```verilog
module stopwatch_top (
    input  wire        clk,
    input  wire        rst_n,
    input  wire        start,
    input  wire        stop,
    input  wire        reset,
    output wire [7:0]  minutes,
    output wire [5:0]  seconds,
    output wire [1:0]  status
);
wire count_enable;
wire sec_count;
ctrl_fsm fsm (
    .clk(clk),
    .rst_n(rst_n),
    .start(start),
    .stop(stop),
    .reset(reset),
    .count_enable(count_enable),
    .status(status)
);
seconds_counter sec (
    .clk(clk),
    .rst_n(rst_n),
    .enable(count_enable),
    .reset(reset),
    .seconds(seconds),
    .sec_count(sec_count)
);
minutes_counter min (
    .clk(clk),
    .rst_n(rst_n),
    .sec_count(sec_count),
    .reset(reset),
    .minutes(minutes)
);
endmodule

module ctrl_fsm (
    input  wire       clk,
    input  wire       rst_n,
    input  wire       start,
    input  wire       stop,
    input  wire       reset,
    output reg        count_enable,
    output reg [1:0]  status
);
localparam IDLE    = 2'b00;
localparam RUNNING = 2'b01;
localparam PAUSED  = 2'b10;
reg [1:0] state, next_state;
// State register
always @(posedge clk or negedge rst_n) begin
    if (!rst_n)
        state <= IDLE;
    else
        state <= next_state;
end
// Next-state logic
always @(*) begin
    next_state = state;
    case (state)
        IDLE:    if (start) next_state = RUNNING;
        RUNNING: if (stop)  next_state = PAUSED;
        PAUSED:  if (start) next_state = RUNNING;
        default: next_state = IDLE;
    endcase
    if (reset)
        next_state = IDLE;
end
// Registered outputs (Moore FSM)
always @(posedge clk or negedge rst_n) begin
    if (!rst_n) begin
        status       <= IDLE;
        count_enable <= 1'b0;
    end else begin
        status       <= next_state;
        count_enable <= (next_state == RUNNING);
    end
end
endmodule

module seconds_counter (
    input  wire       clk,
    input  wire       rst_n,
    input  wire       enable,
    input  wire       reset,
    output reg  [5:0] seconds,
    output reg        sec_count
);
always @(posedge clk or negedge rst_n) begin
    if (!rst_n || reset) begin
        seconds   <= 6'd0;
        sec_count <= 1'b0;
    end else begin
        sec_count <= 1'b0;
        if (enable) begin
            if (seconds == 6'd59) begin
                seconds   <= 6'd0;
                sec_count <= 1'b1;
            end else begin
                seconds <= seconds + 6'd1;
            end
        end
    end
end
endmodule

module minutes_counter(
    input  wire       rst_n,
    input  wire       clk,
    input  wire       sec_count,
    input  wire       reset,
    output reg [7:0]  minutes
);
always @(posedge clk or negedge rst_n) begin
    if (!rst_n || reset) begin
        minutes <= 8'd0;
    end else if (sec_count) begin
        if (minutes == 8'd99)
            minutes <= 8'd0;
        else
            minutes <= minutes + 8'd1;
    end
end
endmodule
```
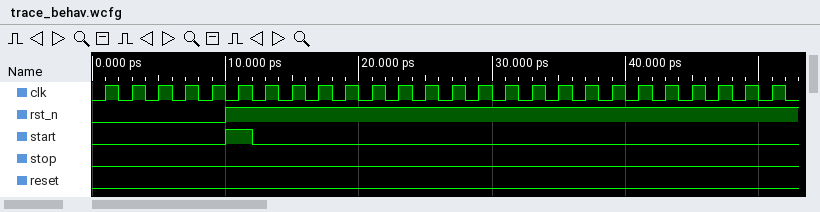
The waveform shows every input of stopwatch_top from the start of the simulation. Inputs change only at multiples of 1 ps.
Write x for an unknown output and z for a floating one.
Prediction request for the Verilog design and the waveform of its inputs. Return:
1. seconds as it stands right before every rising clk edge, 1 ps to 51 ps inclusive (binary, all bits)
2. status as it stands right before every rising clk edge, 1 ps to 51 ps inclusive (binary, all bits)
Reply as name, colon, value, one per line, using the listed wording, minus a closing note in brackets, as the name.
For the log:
seconds as it stands right before every rising clk edge, 1 ps to 51 ps inclusive: 000000, 000000, 000000, 000000, 000000, 000000, 000000, 000001, 000010, 000011, 000100, 000101, 000110, 000111, 001000, 001001, 001010, 001011, 001100, 001101, 001110, 001111, 010000, 010001, 010010, 010011
status as it stands right before every rising clk edge, 1 ps to 51 ps inclusive: 00, 00, 00, 00, 00, 00, 01, 01, 01, 01, 01, 01, 01, 01, 01, 01, 01, 01, 01, 01, 01, 01, 01, 01, 01, 01
